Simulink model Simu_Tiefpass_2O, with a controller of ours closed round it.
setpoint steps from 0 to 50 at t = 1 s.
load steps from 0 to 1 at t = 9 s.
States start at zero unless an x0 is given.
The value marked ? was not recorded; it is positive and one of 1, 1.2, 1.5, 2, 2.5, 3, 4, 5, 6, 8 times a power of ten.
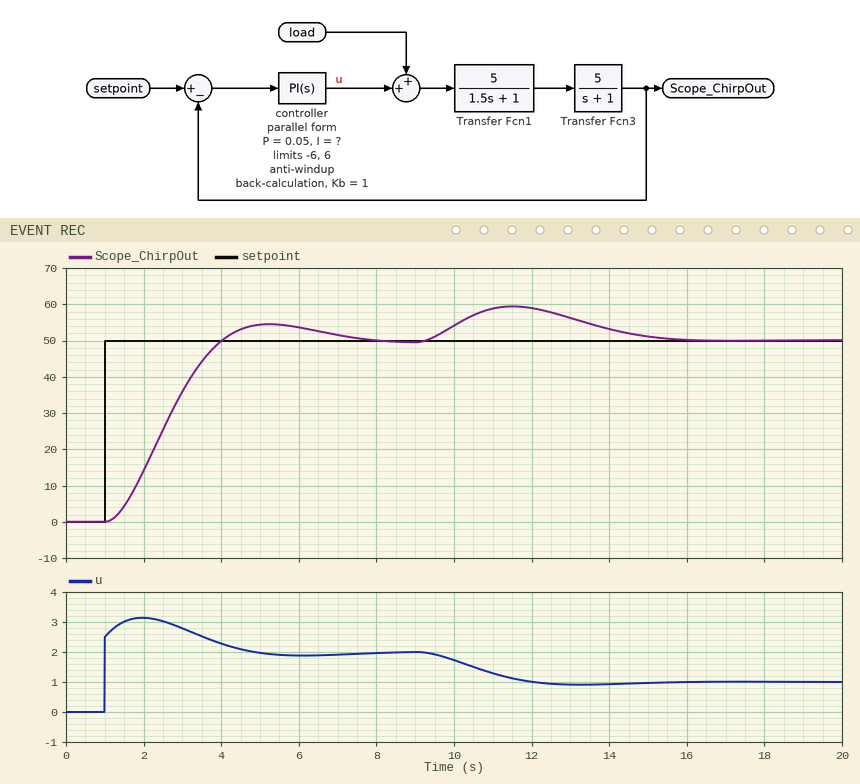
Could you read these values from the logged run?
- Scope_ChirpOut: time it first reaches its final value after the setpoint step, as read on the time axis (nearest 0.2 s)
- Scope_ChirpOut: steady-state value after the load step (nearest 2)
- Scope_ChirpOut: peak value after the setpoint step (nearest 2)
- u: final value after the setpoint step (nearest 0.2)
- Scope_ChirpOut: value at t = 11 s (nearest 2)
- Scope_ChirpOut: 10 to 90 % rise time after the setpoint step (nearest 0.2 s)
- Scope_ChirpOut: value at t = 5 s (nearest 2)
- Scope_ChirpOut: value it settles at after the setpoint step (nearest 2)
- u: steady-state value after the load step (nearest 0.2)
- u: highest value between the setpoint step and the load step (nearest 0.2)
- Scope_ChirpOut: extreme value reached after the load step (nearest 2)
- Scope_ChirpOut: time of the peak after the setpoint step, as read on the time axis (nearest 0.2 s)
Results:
4.0 s
50
54
2.0
58
2.0 s
54
50
1.0
3.2
60
5.2 s
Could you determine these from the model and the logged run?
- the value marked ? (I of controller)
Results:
0.03
